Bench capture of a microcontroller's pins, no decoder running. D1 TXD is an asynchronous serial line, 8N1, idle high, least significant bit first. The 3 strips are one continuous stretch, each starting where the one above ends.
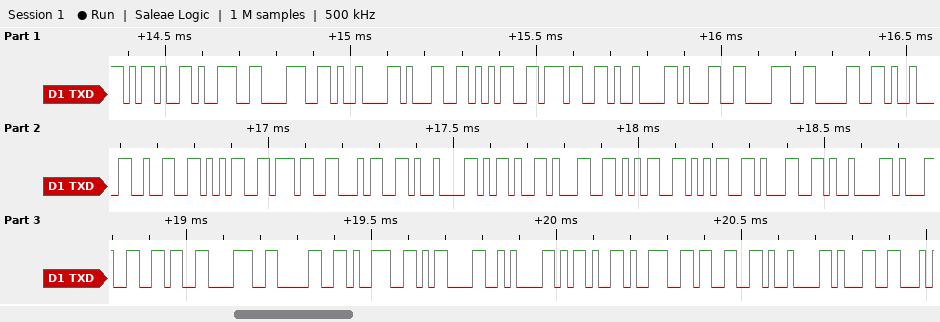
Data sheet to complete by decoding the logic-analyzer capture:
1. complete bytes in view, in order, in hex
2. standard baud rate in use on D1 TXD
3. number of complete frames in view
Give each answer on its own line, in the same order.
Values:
2D 39 38 09 31 35 37 09 31 38 30 09 32 35 37 34 09 2D 31 35 35 31 09 31 36 38 30 39 0D 0A 2D 39 33 09 31
57600 baud
35
